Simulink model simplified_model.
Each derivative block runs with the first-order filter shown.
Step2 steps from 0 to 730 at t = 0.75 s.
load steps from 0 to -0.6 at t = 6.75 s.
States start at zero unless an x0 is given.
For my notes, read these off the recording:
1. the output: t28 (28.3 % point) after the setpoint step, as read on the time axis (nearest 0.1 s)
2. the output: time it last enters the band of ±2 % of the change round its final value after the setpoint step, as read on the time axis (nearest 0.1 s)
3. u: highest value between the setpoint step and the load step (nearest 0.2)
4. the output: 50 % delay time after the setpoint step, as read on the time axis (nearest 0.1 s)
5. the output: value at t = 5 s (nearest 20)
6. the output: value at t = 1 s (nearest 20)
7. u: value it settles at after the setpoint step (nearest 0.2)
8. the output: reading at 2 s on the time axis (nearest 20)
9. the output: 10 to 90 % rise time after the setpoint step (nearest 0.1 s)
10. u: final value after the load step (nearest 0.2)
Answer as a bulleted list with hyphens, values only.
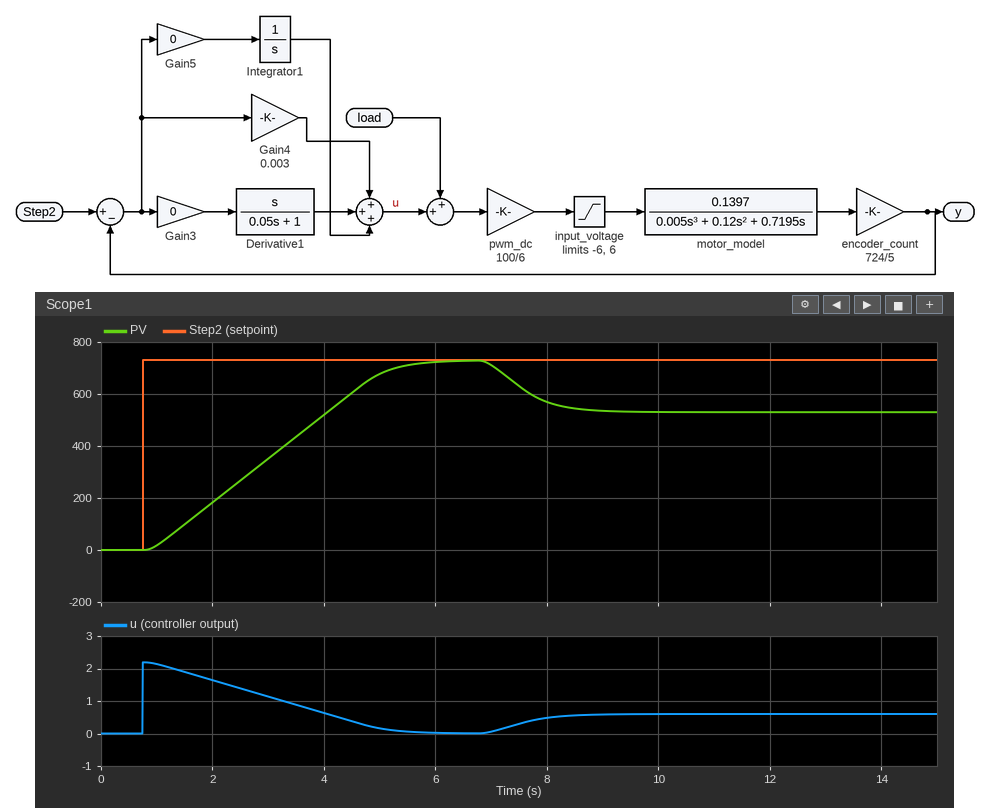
- 2.1 s
- 5.6 s
- 2.2
- 3.1 s
- 680
- 20
- 0.0
- 180
- 3.5 s
- 0.6
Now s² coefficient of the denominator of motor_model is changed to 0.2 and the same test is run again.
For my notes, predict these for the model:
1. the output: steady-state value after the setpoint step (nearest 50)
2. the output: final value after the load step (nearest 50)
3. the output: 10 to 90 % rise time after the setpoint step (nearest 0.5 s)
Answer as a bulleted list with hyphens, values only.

- 750
- 550
- 3.5 s
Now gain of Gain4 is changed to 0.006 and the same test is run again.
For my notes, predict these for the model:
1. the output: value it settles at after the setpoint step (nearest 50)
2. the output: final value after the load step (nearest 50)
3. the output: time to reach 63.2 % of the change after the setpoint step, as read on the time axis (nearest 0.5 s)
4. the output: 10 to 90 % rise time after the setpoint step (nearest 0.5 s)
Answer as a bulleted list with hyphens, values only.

- 750
- 650
- 3.5 s
- 3.5 s
